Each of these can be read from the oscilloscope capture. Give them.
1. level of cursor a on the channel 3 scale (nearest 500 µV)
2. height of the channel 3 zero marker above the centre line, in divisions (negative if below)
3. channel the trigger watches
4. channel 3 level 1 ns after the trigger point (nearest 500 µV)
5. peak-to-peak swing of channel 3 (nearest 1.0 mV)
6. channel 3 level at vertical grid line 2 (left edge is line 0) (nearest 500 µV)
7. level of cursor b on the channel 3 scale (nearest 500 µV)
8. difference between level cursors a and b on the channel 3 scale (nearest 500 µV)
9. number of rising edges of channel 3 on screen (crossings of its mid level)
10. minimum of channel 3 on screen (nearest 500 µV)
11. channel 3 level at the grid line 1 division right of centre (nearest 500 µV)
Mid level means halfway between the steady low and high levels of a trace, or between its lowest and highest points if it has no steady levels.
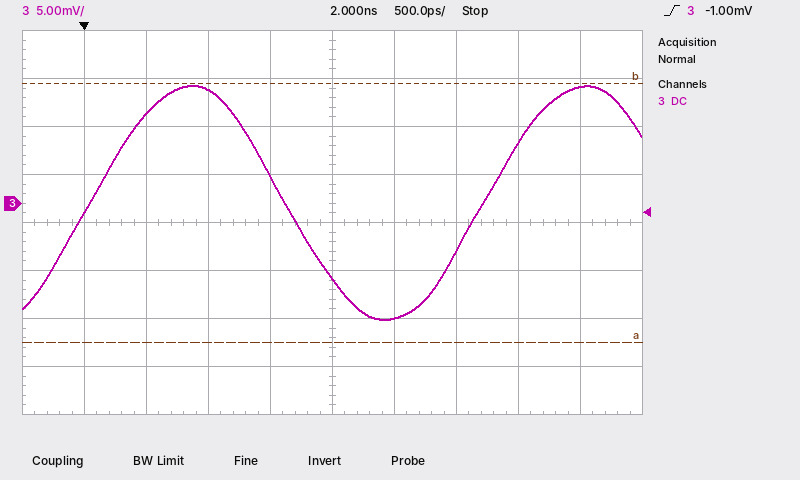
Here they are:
-14.5 mV
+0.4 div
channel 3
12.0 mV
24.0 mV
9.5 mV
12.5 mV
27.0 mV
2
-12.0 mV
-12.0 mV
